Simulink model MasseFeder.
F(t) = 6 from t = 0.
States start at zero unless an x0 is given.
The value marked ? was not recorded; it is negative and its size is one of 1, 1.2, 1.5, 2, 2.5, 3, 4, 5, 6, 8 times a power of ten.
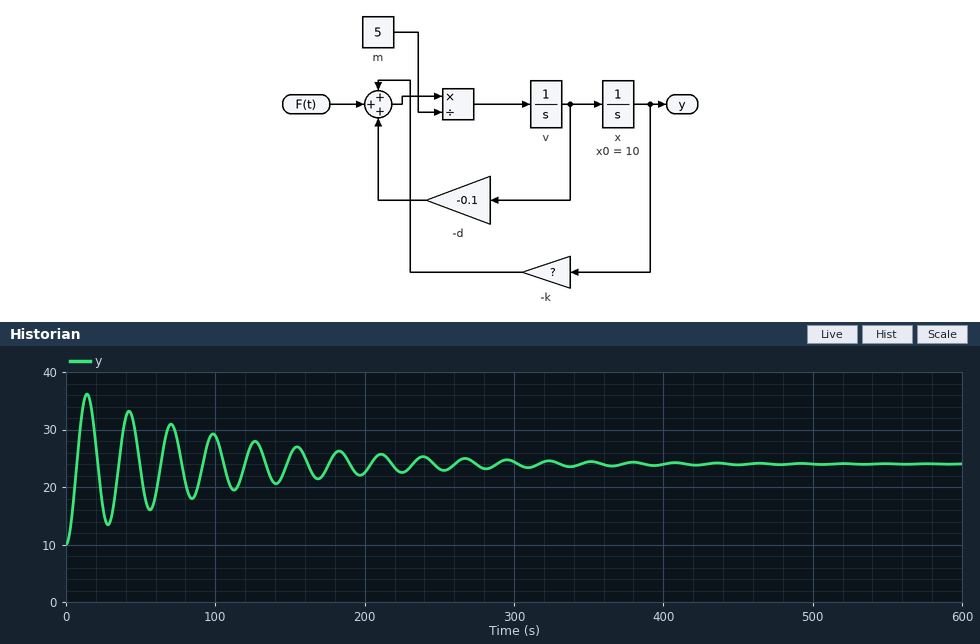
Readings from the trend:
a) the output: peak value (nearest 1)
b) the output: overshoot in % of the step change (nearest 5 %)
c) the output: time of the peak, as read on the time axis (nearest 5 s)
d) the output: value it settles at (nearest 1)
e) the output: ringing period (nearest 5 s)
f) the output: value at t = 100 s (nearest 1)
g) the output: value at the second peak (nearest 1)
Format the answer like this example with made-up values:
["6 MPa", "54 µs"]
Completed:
["36", "85 %", "15 s", "24", "30 s", "29", "33"]
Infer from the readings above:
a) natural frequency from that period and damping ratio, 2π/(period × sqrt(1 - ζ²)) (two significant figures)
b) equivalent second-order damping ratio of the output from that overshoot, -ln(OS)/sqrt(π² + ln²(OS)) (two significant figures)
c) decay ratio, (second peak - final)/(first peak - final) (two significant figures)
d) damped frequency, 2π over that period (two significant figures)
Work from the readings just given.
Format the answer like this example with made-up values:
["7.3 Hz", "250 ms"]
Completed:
["0.21 rad/s", "0.052", "0.75", "0.21 rad/s"]
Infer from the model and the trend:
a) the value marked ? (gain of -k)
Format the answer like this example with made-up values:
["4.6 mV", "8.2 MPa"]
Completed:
["-0.25"]
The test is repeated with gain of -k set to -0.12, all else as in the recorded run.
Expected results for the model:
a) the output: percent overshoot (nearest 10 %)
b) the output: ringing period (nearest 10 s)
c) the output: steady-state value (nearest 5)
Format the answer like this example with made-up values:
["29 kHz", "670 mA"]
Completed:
["80 %", "40 s", "50"]
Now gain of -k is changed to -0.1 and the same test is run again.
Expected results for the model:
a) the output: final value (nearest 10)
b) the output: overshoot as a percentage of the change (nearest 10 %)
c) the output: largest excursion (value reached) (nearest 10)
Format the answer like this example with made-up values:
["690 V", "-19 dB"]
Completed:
["60", "80 %", "100"]
